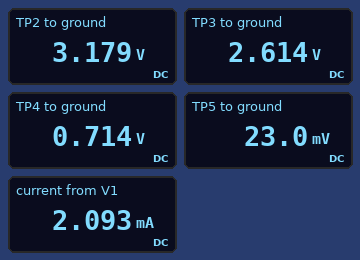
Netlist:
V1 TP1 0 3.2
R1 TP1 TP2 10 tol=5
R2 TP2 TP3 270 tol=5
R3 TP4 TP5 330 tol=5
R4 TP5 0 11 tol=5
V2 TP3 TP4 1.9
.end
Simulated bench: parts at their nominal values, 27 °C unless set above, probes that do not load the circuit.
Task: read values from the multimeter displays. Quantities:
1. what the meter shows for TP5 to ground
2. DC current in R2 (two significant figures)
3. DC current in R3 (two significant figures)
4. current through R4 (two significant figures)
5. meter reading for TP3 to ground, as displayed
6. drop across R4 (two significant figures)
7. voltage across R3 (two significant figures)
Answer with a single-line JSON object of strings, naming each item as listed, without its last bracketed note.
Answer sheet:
{"what the meter shows for TP5 to ground": "23.0 mV", "DC current in R2": "2.1 mA", "DC current in R3": "2.1 mA", "current through R4": "2.1 mA", "meter reading for TP3 to ground, as displayed": "2.614 V", "drop across R4": "23 mV", "voltage across R3": "690 mV"}
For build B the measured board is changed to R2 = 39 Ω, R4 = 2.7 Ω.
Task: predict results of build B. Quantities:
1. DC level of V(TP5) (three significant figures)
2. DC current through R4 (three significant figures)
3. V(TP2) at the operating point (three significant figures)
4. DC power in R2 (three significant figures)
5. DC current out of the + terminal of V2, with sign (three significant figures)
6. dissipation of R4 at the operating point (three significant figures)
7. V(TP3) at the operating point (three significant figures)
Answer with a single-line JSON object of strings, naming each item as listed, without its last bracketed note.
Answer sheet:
{"DC level of V(TP5)": "9.20 mV", "DC current through R4": "3.41 mA", "V(TP2) at the operating point": "3.17 V", "DC power in R2": "452 µW", "DC current out of the + terminal of V2, with sign": "-3.41 mA", "dissipation of R4 at the operating point": "31.3 µW", "V(TP3) at the operating point": "3.03 V"}
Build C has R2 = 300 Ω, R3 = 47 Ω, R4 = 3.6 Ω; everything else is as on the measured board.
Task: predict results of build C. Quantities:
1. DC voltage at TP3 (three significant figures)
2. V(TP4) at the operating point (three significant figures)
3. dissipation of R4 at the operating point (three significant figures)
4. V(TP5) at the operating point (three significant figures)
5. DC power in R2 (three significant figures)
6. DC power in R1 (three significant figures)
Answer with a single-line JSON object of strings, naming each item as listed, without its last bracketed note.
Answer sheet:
{"DC voltage at TP3": "2.08 V", "V(TP4) at the operating point": "182 mV", "dissipation of R4 at the operating point": "46.8 µW", "V(TP5) at the operating point": "13.0 mV", "DC power in R2": "3.90 mW", "DC power in R1": "130 µW"}
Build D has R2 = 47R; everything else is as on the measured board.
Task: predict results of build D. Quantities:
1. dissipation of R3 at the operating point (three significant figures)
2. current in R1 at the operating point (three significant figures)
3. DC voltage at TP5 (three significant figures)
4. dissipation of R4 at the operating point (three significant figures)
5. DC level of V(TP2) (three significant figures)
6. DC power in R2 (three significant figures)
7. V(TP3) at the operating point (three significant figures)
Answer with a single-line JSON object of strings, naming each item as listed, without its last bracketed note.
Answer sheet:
{"dissipation of R3 at the operating point": "3.52 mW", "current in R1 at the operating point": "3.27 mA", "DC voltage at TP5": "35.9 mV", "dissipation of R4 at the operating point": "117 µW", "DC level of V(TP2)": "3.17 V", "DC power in R2": "501 µW", "V(TP3) at the operating point": "3.01 V"}
